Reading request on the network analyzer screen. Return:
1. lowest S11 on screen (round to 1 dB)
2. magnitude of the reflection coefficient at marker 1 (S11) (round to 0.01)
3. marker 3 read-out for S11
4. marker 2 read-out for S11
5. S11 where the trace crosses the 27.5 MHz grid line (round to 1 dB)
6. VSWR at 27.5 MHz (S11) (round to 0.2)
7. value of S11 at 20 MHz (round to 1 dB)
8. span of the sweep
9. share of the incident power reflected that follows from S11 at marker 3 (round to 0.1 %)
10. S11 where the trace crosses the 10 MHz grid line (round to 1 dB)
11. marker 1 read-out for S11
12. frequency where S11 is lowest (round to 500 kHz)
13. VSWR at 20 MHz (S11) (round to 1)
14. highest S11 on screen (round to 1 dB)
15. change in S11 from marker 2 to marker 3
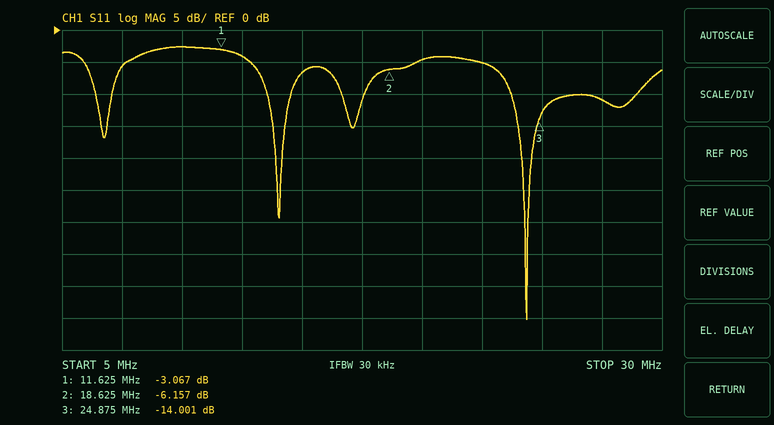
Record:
-45 dB
0.70
-14.001 dB
-6.157 dB
-11 dB
1.8
-5 dB
25 MHz
4.0 %
-3 dB
-3.067 dB
24.5 MHz
4
-3 dB
-7.844 dB
